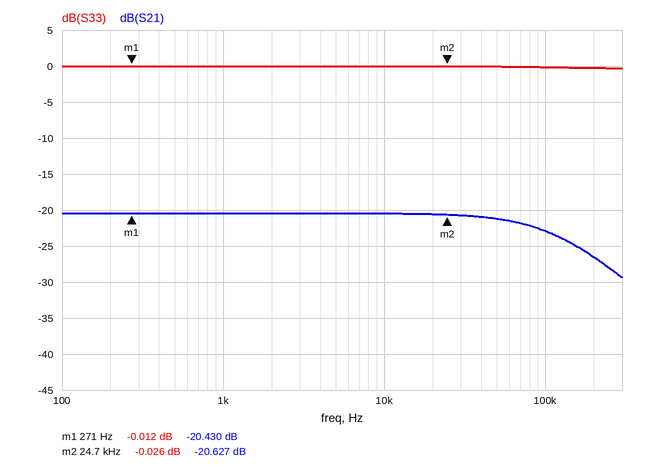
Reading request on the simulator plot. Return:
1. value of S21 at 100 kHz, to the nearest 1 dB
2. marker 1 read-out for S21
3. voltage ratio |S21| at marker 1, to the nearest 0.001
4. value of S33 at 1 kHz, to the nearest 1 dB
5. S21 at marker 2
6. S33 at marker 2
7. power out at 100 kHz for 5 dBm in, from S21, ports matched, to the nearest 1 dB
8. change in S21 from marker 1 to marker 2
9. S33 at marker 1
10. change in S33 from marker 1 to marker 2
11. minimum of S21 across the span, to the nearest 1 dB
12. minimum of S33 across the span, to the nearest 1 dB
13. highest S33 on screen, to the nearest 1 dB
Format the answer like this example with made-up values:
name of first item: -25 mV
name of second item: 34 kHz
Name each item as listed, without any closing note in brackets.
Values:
value of S21 at 100 kHz, to the nearest 1 dB: -23 dB
marker 1 read-out for S21: -20.430 dB
voltage ratio |S21| at marker 1, to the nearest 0.001: 0.095
value of S33 at 1 kHz, to the nearest 1 dB: 0 dB
S21 at marker 2: -20.627 dB
S33 at marker 2: -0.026 dB
power out at 100 kHz for 5 dBm in, from S21, ports matched, to the nearest 1 dB: -18 dBm
change in S21 from marker 1 to marker 2: -0.197 dB
S33 at marker 1: -0.012 dB
change in S33 from marker 1 to marker 2: -0.014 dB
minimum of S21 across the span, to the nearest 1 dB: -29 dB
minimum of S33 across the span, to the nearest 1 dB: 0 dB
highest S33 on screen, to the nearest 1 dB: 0 dB
